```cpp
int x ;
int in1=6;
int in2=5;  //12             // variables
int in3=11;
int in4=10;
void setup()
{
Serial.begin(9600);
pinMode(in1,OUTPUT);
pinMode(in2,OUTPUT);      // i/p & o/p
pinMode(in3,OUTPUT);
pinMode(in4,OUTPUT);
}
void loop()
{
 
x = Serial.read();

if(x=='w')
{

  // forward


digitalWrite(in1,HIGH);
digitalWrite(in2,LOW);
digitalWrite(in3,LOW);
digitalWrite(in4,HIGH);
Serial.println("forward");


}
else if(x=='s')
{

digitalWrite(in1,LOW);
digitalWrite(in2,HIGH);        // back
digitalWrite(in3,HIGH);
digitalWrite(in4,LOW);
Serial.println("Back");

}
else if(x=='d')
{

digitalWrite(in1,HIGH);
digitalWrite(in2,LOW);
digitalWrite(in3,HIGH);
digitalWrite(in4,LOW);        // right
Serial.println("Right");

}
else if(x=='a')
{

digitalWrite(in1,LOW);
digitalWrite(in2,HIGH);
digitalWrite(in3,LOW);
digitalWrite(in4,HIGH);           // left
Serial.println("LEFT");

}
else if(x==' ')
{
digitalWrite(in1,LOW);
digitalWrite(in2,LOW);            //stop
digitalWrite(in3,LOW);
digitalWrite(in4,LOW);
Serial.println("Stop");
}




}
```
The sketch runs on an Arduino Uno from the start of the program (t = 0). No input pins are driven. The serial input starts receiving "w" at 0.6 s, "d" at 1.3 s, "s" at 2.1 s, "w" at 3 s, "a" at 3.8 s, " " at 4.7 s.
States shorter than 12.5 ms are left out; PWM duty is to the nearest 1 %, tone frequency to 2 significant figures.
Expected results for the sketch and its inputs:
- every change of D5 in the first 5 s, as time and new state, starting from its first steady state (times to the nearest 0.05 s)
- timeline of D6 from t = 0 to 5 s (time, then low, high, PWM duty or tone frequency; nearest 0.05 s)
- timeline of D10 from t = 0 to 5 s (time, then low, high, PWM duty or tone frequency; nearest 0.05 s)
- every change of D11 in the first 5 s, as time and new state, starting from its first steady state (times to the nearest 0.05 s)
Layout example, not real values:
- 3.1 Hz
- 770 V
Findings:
- 0 s low; 2.1 s high; 3 s low; 3.8 s high; 4.7 s low
- 0 s low; 0.6 s high; 2.1 s low; 3 s high; 3.8 s low
- 0 s low; 0.6 s high; 1.3 s low; 3 s high; 4.7 s low
- 0 s low; 1.3 s high; 3 s low
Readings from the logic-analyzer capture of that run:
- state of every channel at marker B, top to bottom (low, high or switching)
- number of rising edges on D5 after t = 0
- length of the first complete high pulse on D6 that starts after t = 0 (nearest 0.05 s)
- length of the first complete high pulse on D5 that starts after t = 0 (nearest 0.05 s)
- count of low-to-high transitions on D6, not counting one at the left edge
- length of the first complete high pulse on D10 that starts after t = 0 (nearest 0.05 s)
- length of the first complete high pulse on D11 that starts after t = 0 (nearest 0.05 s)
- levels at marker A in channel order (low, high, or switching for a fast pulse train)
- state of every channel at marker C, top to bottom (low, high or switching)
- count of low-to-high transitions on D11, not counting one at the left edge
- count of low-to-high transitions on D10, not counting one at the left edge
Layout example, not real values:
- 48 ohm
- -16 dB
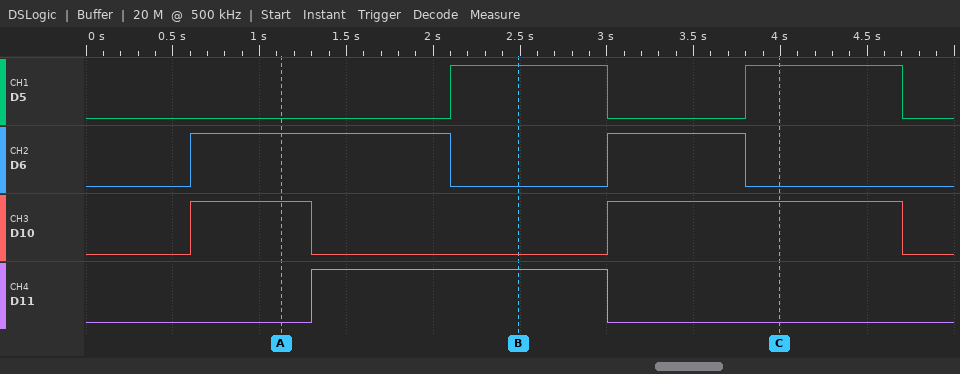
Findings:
- D5 high, D6 low, D10 low, D11 high
- 2
- 1.50 s
- 0.90 s
- 2
- 0.70 s
- 1.70 s
- D5 low, D6 high, D10 high, D11 low
- D5 high, D6 low, D10 high, D11 low
- 1
- 2
